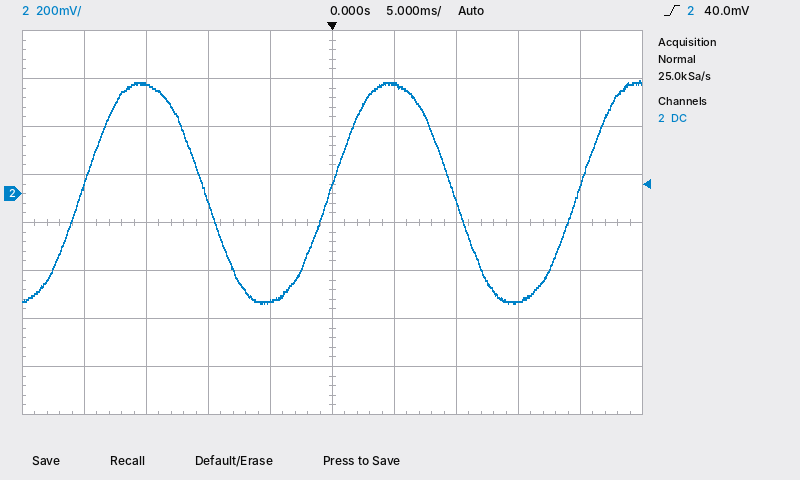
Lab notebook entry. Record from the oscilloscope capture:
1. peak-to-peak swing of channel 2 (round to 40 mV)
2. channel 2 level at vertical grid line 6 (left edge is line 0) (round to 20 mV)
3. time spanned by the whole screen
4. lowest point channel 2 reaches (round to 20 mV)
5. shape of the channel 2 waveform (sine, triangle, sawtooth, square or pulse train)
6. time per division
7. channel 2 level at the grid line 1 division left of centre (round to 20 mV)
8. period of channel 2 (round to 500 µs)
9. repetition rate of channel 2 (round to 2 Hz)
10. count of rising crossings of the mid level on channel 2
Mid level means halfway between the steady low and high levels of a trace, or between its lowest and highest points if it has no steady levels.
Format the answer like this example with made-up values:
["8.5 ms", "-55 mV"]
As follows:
["920 mV", "460 mV", "50 ms", "-460 mV", "sine", "5 ms", "-440 mV", "20.0 ms", "50 Hz", "3"]
